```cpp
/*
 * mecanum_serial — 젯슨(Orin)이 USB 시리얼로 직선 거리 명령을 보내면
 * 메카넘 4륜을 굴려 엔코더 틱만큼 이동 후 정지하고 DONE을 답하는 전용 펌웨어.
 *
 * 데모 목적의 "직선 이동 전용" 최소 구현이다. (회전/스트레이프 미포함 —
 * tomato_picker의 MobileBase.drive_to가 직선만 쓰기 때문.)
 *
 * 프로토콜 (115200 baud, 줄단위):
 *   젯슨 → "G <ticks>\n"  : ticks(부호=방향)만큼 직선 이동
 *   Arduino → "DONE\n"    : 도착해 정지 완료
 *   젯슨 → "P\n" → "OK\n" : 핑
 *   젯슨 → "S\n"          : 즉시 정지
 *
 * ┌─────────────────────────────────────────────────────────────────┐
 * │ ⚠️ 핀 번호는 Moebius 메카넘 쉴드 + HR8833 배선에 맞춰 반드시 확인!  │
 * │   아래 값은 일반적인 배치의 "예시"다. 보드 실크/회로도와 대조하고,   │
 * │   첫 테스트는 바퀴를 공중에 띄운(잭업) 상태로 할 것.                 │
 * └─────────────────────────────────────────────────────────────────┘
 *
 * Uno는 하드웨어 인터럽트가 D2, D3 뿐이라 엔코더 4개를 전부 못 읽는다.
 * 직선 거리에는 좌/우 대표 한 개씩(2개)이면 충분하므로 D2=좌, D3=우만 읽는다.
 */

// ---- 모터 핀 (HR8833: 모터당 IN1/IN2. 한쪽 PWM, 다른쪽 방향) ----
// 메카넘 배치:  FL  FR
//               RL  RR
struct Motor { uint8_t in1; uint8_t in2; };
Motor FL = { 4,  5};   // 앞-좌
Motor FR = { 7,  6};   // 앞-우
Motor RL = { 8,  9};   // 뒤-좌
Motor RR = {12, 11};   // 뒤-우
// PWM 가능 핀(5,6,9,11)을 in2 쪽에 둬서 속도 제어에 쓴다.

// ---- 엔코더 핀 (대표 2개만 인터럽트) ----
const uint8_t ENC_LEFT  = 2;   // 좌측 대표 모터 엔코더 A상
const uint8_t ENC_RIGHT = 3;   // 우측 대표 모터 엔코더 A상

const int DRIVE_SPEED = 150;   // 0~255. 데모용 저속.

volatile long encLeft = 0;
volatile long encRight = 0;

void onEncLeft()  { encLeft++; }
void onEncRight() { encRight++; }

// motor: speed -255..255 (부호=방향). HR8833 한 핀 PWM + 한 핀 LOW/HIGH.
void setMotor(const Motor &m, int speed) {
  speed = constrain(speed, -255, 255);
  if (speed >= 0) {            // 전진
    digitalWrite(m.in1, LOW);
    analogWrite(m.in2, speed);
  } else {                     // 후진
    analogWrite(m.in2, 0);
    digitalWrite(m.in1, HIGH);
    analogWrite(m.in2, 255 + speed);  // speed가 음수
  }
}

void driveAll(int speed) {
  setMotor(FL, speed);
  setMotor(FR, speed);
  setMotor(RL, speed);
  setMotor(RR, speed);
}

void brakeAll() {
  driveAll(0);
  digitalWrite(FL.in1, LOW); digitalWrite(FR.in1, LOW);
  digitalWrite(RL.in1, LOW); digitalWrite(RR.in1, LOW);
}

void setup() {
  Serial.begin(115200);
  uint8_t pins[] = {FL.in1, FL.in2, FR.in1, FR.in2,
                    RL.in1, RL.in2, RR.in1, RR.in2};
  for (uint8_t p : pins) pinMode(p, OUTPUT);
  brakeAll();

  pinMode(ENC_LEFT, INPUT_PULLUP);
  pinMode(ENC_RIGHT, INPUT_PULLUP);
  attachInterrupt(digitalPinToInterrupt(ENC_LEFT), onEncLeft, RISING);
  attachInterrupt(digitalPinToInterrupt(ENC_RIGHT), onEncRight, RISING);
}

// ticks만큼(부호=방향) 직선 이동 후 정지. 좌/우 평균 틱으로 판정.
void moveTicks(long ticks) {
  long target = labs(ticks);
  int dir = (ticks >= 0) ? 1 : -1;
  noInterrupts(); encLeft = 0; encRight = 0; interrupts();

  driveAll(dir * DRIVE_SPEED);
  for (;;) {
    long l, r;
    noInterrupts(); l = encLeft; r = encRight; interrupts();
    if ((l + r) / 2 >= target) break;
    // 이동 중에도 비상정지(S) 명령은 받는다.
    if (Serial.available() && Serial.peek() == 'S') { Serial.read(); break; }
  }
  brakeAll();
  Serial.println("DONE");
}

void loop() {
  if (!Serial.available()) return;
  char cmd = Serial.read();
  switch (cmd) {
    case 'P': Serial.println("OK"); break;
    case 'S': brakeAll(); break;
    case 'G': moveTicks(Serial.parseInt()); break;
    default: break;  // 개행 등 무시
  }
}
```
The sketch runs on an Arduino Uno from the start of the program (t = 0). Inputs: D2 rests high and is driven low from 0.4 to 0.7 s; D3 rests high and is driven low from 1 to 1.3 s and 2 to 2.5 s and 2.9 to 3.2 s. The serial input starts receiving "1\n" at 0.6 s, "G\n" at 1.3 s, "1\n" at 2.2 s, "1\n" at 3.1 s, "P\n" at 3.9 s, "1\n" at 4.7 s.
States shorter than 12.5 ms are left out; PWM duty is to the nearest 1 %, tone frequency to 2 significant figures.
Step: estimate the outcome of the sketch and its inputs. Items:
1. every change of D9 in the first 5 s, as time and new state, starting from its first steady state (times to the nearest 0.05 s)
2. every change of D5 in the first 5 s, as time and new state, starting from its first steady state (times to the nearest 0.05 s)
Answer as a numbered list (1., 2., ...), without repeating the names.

1. 0 s low; 2.2 s PWM 59 %; 3.2 s low
2. 0 s low; 2.2 s PWM 59 %; 3.2 s low
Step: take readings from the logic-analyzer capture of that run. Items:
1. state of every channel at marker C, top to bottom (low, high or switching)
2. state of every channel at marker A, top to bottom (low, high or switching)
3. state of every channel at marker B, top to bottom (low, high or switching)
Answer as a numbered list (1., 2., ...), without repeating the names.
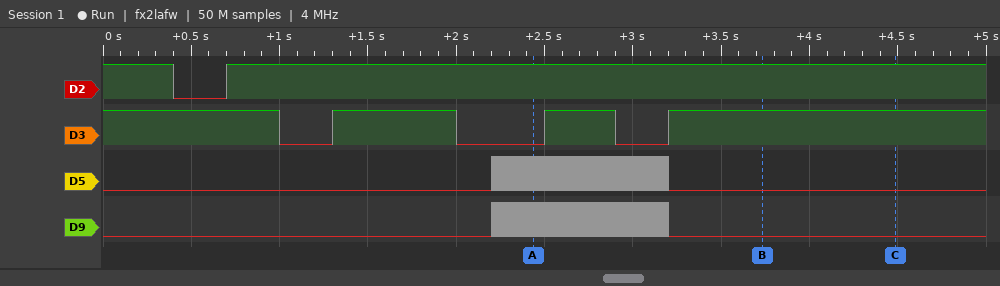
1. D2 high, D3 high, D5 low, D9 low
2. D2 high, D3 low, D5 switching, D9 switching
3. D2 high, D3 high, D5 low, D9 low
